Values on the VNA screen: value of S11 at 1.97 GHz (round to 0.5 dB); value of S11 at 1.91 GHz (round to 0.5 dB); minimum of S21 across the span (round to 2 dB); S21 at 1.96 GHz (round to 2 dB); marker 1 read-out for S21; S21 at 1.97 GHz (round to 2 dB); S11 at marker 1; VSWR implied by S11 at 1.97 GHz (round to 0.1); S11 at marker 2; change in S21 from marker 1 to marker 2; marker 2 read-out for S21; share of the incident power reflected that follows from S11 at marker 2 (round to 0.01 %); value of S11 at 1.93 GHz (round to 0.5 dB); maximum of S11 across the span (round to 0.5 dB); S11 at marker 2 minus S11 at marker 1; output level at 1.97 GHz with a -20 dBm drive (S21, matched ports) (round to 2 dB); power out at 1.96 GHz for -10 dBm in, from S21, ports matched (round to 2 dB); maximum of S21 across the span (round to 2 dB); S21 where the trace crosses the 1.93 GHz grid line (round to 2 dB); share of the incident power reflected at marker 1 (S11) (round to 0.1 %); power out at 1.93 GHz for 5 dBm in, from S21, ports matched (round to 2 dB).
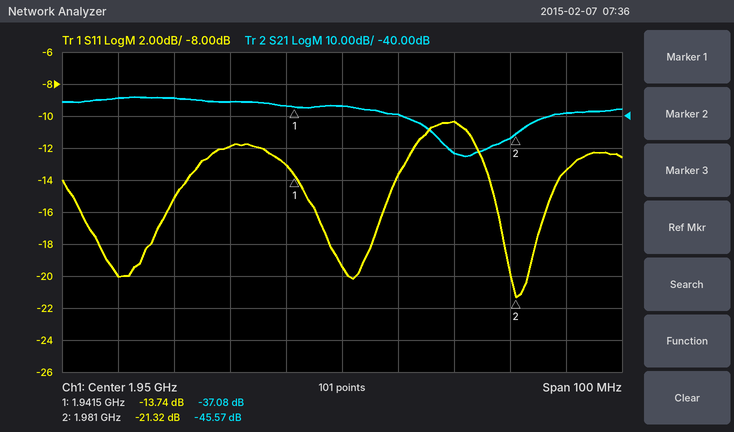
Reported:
-10.5 dB
-20.0 dB
-52 dB
-40 dB
-37.08 dB
-52 dB
-13.74 dB
1.9
-21.32 dB
-8.49 dB
-45.57 dB
0.74 %
-12.0 dB
-10.5 dB
-7.58 dB
-72 dBm
-50 dBm
-34 dB
-36 dB
4.2 %
-30 dBm
